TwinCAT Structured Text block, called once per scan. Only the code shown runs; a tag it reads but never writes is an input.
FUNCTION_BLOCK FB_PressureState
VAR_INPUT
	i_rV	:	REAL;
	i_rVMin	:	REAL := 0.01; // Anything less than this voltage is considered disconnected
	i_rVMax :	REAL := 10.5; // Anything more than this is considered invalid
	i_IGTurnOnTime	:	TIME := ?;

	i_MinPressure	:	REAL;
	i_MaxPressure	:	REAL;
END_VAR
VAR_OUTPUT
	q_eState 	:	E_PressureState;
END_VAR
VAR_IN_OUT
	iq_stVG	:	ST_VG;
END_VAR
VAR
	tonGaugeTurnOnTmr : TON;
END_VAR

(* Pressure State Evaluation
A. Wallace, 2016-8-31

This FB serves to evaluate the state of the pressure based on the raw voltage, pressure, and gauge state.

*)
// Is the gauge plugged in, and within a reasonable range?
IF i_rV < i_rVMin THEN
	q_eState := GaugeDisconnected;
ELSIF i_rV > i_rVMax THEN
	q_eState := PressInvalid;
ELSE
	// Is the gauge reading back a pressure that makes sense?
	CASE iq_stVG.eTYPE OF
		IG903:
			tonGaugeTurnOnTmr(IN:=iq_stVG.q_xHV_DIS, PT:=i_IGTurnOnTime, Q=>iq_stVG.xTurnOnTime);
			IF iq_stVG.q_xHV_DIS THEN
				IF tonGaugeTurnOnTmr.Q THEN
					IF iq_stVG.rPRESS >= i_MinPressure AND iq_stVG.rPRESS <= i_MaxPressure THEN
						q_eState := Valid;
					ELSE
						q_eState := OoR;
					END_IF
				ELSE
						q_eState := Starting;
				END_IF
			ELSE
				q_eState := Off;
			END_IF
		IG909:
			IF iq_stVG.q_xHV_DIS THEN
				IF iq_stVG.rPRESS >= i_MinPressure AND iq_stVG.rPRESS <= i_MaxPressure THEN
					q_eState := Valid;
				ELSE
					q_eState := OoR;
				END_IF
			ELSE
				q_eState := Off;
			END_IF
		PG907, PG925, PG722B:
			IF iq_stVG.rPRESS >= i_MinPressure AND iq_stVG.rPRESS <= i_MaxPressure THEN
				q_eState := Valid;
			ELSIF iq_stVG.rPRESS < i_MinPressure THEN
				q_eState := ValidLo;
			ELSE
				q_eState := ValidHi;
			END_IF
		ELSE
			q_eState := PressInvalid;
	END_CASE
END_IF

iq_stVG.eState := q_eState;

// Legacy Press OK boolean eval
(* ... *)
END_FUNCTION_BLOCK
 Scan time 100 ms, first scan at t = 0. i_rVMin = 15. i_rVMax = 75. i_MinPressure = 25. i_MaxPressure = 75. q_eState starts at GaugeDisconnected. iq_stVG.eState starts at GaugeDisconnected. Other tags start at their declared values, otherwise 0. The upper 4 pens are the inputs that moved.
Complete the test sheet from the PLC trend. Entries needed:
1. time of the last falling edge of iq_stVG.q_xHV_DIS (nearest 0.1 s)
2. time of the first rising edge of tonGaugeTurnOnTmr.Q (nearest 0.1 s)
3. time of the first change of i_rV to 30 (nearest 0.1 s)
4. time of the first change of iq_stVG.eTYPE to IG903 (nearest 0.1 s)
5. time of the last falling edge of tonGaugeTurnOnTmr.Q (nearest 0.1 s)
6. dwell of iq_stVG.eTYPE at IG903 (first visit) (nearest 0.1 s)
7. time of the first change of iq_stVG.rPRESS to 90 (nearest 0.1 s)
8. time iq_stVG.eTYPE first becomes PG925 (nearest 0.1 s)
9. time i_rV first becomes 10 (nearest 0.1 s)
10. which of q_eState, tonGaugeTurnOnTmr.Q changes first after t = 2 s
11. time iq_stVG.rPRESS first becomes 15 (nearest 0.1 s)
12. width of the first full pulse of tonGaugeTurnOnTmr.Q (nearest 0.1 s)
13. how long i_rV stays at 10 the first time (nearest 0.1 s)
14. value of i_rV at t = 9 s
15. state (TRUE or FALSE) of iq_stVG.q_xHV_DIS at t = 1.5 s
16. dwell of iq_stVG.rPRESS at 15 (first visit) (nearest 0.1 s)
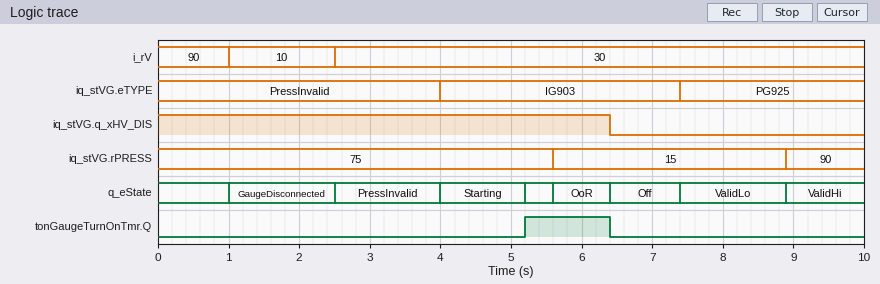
6.4 s
5.2 s
2.5 s
4.0 s
6.4 s
3.4 s
8.9 s
7.4 s
1.0 s
q_eState
5.6 s
1.2 s
1.5 s
30
TRUE
3.3 s
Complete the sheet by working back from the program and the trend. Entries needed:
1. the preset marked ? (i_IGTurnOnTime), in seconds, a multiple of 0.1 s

1.2 s
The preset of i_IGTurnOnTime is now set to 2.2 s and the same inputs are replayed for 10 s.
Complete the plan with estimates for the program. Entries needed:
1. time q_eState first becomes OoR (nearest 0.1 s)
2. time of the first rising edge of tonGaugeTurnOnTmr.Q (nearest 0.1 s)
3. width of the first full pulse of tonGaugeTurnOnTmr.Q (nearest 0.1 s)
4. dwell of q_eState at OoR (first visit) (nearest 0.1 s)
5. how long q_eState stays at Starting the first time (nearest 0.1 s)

6.2 s
6.2 s
0.2 s
0.2 s
2.2 s
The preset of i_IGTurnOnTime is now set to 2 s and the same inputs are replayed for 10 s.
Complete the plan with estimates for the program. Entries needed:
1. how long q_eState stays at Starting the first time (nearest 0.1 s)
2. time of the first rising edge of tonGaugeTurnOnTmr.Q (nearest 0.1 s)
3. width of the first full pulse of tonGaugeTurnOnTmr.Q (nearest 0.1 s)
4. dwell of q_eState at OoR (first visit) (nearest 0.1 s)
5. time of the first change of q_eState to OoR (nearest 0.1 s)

2.0 s
6.0 s
0.4 s
0.4 s
6.0 s
